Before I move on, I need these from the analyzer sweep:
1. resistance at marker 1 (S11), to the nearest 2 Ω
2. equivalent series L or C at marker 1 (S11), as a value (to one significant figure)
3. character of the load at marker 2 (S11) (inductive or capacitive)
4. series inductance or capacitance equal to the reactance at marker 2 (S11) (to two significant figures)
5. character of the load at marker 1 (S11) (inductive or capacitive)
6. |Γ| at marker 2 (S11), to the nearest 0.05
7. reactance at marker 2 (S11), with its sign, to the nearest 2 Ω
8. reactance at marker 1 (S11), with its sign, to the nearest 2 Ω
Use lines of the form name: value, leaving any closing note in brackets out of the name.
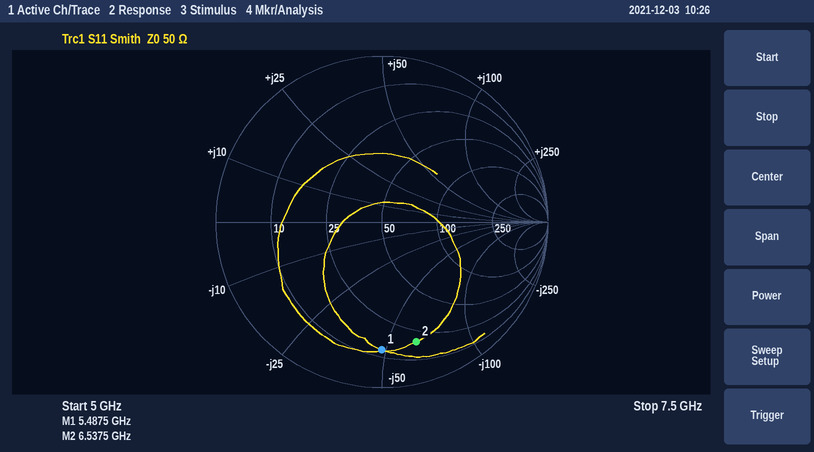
resistance at marker 1 (S11), to the nearest 2 Ω: 12 Ω
equivalent series L or C at marker 1 (S11), as a value: 600 fF
character of the load at marker 2 (S11): capacitive
series inductance or capacitance equal to the reactance at marker 2 (S11): 390 fF
character of the load at marker 1 (S11): capacitive
|Γ| at marker 2 (S11), to the nearest 0.05: 0.75
reactance at marker 2 (S11), with its sign, to the nearest 2 Ω: -62 Ω
reactance at marker 1 (S11), with its sign, to the nearest 2 Ω: -48 Ω
